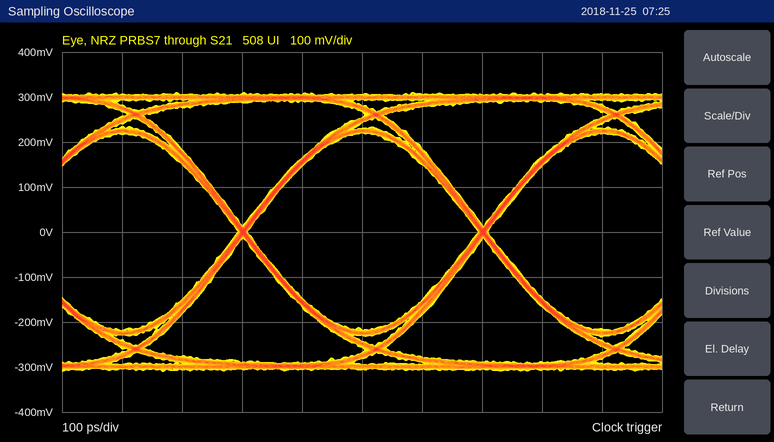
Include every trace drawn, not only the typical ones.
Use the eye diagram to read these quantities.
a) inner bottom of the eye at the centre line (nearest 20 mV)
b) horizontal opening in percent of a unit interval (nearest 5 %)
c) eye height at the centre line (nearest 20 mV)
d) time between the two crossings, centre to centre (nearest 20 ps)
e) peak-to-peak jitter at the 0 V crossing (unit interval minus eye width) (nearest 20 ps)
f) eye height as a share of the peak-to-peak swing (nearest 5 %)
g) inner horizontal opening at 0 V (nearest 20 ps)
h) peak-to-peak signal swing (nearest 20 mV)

-220 mV
95 %
440 mV
400 ps
20 ps
70 %
380 ps
620 mV
